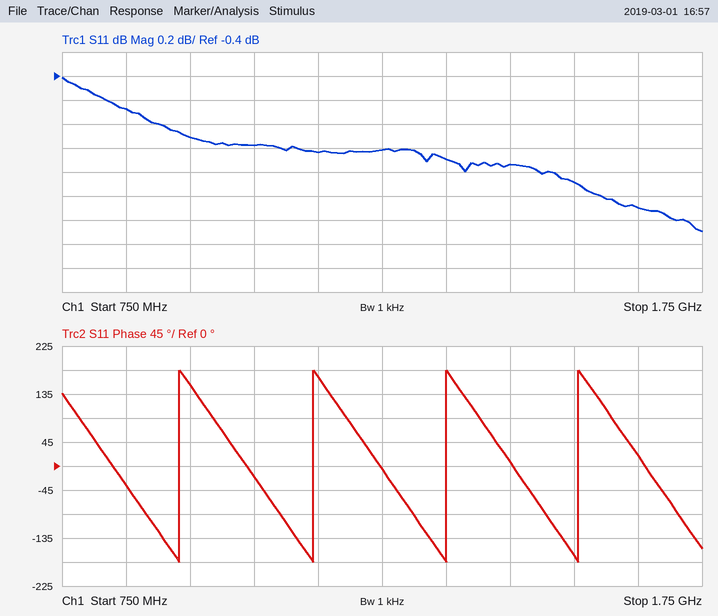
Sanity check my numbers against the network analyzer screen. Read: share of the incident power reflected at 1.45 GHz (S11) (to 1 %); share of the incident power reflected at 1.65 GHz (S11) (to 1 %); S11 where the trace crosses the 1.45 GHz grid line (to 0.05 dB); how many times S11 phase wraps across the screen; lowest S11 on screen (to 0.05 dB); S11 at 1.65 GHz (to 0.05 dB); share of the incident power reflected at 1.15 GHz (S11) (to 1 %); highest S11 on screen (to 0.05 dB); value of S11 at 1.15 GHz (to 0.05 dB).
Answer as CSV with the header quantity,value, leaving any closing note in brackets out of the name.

quantity,value
share of the incident power reflected at 1.45 GHz (S11),77 %
share of the incident power reflected at 1.65 GHz (S11),71 %
S11 where the trace crosses the 1.45 GHz grid line,-1.15 dB
how many times S11 phase wraps across the screen,4
lowest S11 on screen,-1.70 dB
S11 at 1.65 GHz,-1.50 dB
share of the incident power reflected at 1.15 GHz (S11),79 %
highest S11 on screen,-0.40 dB
value of S11 at 1.15 GHz,-1.05 dB
